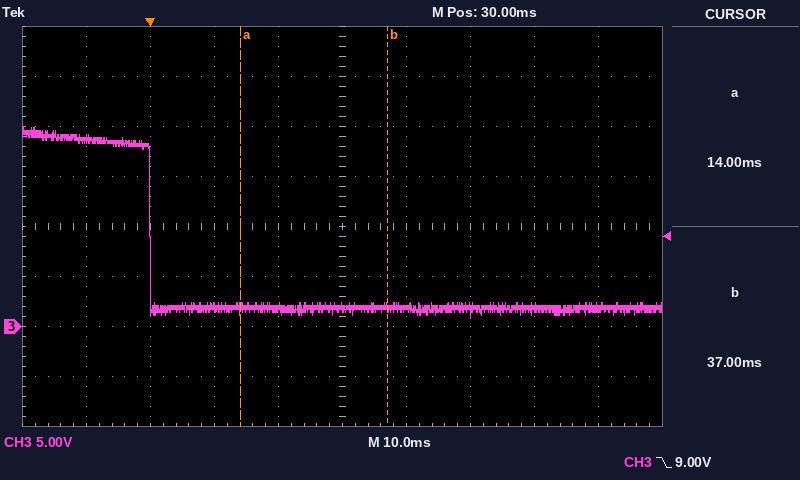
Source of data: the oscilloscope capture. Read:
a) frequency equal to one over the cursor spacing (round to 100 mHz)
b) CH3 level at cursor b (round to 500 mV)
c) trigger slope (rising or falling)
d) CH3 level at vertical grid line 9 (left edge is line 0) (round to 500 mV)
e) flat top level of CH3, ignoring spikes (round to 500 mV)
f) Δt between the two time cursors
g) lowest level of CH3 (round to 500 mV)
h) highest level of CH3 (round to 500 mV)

43.5 Hz
2.0 V
falling
2.0 V
18.5 V
23 ms
1.0 V
20.0 V
